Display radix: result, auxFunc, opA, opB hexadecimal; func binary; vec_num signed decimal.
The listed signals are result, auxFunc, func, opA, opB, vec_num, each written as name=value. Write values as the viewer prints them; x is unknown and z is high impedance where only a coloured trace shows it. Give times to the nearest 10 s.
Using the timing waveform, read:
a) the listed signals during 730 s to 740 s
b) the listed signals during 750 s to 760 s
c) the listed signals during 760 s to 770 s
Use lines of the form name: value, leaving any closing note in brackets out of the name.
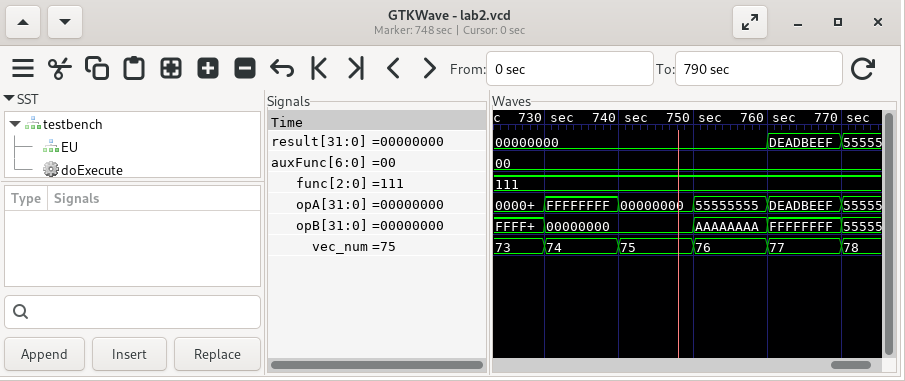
the listed signals during 730 s to 740 s: result=00000000, auxFunc=00, func=111, opA=FFFFFFFF, opB=00000000, vec_num=74
the listed signals during 750 s to 760 s: result=00000000, auxFunc=00, func=111, opA=55555555, opB=AAAAAAAA, vec_num=76
the listed signals during 760 s to 770 s: result=DEADBEEF, auxFunc=00, func=111, opA=DEADBEEF, opB=FFFFFFFF, vec_num=77
